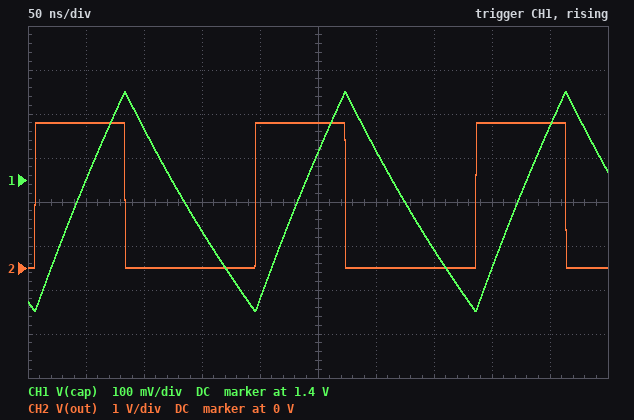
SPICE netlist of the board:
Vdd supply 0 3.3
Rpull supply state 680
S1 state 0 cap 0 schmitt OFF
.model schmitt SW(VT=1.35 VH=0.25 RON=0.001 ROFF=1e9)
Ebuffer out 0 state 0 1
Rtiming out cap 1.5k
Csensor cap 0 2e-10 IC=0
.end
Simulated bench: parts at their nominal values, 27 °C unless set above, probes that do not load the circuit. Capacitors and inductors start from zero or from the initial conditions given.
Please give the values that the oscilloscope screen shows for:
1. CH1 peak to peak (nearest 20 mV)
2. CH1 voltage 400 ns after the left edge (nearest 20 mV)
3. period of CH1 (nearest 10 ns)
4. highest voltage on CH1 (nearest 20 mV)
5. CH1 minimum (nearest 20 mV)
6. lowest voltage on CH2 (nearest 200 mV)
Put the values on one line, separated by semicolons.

500 mV; 1.20 V; 190 ns; 1.60 V; 1.10 V; 0 V
